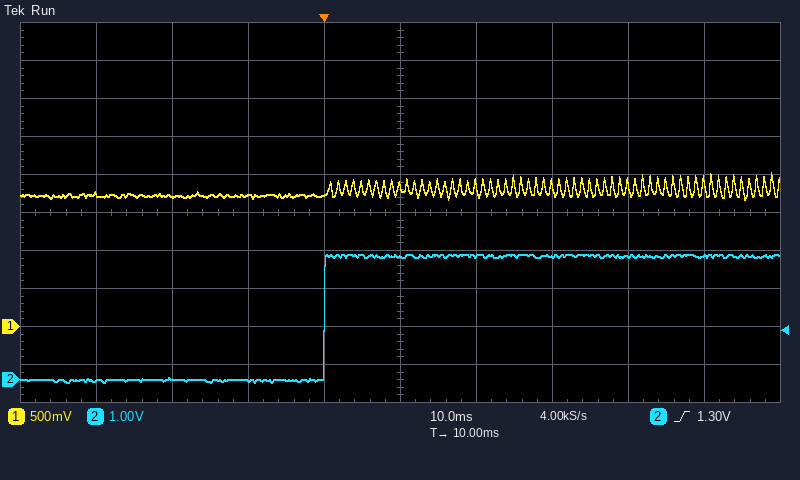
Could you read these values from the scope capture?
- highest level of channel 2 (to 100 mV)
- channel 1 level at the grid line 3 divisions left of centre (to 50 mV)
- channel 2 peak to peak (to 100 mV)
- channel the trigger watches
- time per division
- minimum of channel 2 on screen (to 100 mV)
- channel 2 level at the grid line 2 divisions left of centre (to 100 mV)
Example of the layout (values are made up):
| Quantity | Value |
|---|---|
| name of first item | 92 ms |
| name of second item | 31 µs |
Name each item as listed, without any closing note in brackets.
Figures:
| Quantity | Value |
|---|---|
| highest level of channel 2 | 3.3 V |
| channel 1 level at the grid line 3 divisions left of centre | 1.70 V |
| channel 2 peak to peak | 3.4 V |
| channel the trigger watches | channel 2 |
| time per division | 10 ms |
| minimum of channel 2 on screen | -100 mV |
| channel 2 level at the grid line 2 divisions left of centre | 0.0 V |
